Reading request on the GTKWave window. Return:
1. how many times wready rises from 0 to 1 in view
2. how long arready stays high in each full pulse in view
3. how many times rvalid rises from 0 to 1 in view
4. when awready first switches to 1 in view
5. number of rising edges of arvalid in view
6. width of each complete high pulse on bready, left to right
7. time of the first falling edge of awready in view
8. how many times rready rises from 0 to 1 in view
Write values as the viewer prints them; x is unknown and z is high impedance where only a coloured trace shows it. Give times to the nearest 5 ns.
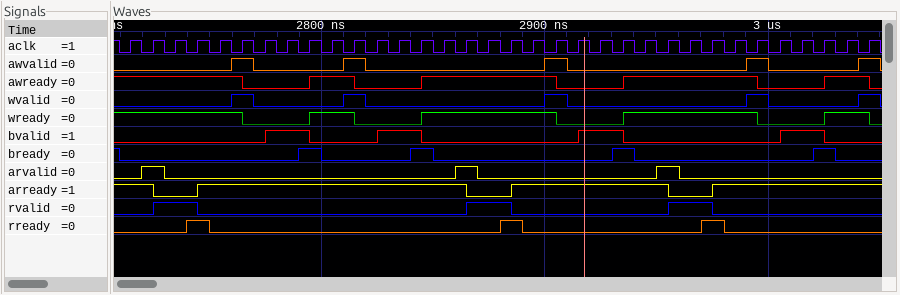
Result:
4
120 ns, 70 ns
3
2795 ns
3
10 ns, 10 ns, 10 ns, 10 ns
2765 ns
3
